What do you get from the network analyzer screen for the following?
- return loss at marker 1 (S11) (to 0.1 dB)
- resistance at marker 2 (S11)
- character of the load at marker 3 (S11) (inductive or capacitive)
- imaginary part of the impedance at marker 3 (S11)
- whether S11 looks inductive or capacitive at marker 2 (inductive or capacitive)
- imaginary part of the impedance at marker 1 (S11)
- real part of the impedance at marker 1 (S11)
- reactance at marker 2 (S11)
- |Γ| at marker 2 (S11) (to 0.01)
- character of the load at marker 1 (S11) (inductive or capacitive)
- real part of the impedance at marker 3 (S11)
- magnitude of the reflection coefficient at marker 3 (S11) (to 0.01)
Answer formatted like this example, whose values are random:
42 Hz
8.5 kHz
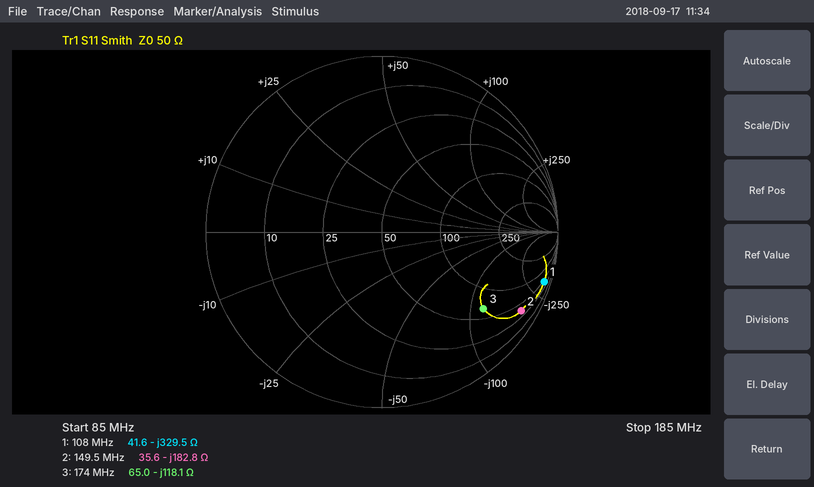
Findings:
0.3 dB
35.6 Ω
capacitive
-118.1 Ω
capacitive
-329.5 Ω
41.6 Ω
-182.8 Ω
0.91
capacitive
65.0 Ω
0.72
